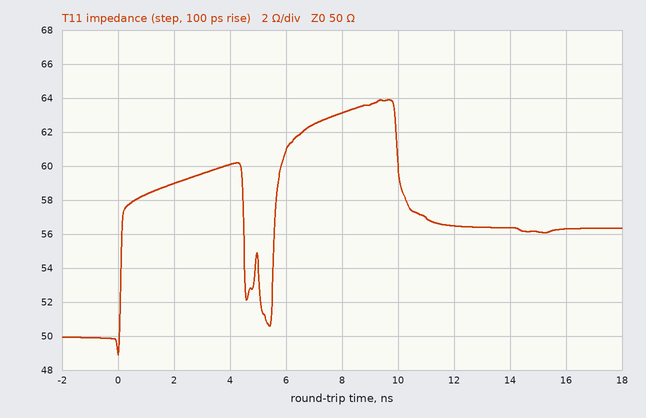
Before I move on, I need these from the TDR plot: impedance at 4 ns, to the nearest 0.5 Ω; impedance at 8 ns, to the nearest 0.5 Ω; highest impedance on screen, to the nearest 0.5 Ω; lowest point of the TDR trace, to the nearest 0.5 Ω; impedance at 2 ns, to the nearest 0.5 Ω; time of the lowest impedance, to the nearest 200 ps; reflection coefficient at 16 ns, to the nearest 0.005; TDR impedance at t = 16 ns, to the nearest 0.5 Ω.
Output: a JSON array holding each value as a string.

["60.0 Ω", "63.0 Ω", "64.0 Ω", "49.0 Ω", "59.0 Ω", "0.0 ns", "+0.060", "56.5 Ω"]
